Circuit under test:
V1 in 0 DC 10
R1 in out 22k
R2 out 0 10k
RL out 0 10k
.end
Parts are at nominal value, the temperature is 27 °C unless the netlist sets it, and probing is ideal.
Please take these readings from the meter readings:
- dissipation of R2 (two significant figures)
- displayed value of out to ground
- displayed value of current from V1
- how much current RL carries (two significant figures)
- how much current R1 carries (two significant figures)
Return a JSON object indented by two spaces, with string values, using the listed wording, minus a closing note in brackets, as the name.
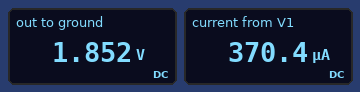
{
  "dissipation of R2": "340 µW",
  "displayed value of out to ground": "1.852 V",
  "displayed value of current from V1": "370.4 µA",
  "how much current RL carries": "190 µA",
  "how much current R1 carries": "370 µA"
}
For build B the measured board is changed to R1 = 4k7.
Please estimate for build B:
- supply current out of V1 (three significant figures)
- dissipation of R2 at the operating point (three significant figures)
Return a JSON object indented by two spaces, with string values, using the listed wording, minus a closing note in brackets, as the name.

{
  "supply current out of V1": "1.03 mA",
  "dissipation of R2 at the operating point": "2.66 mW"
}
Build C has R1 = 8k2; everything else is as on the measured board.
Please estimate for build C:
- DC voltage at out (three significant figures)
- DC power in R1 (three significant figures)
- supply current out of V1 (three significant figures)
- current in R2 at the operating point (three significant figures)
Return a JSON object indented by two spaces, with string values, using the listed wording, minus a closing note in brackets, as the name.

{
  "DC voltage at out": "3.79 V",
  "DC power in R1": "4.71 mW",
  "supply current out of V1": "758 µA",
  "current in R2 at the operating point": "379 µA"
}
